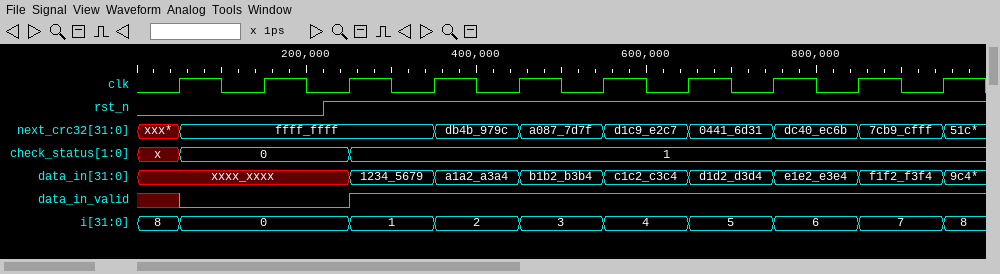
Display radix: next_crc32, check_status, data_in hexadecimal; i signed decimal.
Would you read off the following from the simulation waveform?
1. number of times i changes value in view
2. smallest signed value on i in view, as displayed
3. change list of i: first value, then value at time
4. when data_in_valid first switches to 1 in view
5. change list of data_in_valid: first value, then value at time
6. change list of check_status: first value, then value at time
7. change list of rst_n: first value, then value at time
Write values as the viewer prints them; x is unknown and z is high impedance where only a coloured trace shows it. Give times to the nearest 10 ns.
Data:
9
0
8, 0 at 50 ns, 1 at 250 ns, 2 at 350 ns, 3 at 450 ns, 4 at 550 ns, 5 at 650 ns, 6 at 750 ns, 7 at 850 ns, 8 at 950 ns
250 ns
x, 0 at 50 ns, 1 at 250 ns
x, 0 at 50 ns, 1 at 250 ns
0, 1 at 220 ns
